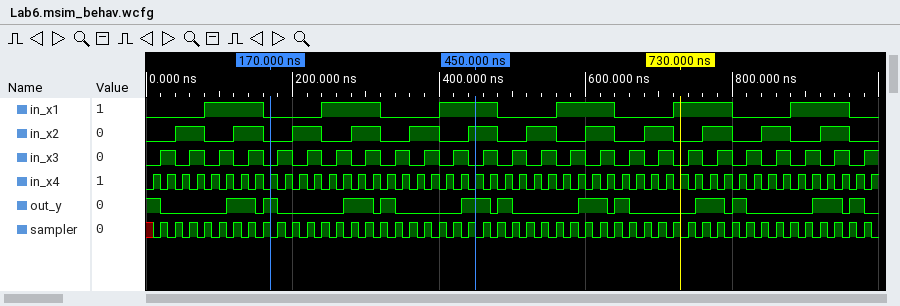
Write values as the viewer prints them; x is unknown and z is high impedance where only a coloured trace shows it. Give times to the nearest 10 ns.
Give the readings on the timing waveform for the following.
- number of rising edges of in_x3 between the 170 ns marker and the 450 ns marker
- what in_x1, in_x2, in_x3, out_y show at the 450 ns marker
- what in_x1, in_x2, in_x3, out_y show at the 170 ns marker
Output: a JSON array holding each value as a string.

["7", "in_x1=1, in_x2=1, in_x3=0, out_y=1", "in_x1=0, in_x2=0, in_x3=0, out_y=1"]
